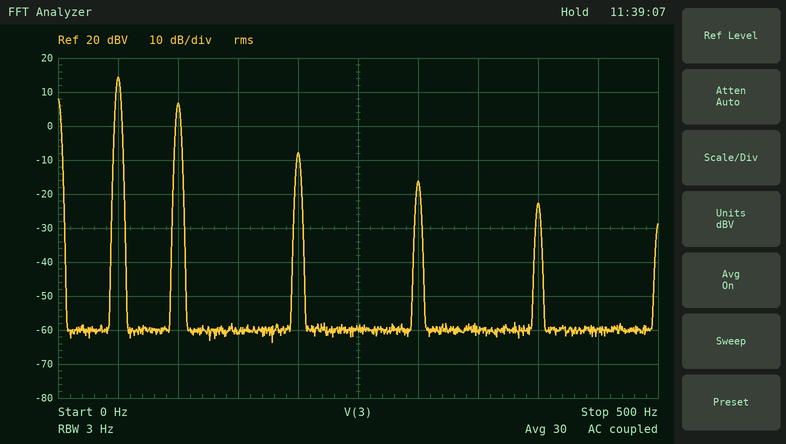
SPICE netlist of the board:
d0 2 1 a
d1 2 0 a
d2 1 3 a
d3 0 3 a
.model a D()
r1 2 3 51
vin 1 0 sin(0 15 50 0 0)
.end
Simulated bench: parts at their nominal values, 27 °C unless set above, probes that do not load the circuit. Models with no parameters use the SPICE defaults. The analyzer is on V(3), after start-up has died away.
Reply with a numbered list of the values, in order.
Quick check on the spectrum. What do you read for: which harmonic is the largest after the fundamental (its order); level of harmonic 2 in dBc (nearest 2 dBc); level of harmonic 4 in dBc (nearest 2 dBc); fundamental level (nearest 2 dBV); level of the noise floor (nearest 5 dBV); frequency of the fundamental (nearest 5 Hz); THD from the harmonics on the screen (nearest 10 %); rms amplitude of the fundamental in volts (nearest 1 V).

1. 2
2. -8 dBc
3. -22 dBc
4. 14 dBV
5. -60 dBV
6. 50 Hz
7. 40 %
8. 5 V
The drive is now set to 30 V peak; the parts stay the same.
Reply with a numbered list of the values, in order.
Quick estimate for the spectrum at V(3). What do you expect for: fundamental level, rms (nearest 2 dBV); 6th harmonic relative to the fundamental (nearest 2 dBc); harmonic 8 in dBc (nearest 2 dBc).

1. 20 dBV
2. -30 dBc
3. -34 dBc
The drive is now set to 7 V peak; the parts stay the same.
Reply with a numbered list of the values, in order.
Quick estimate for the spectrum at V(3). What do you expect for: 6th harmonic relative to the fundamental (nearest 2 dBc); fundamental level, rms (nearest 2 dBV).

1. -38 dBc
2. 8 dBV
